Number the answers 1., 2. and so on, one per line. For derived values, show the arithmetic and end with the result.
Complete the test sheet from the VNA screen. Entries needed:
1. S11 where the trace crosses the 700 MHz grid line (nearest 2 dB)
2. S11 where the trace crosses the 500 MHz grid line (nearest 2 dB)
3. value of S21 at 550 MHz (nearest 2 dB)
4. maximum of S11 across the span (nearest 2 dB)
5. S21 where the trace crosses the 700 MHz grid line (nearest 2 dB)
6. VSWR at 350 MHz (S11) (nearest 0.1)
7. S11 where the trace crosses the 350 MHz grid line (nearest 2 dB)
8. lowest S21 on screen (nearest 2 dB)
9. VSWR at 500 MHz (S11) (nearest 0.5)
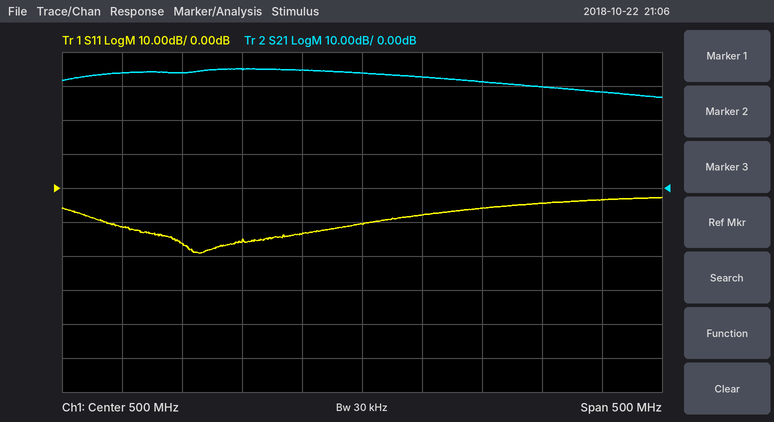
1. -4 dB
2. -10 dB
3. 32 dB
4. -2 dB
5. 28 dB
6. |Γ| = 10^(-16/20) = 0.1585; VSWR = (1 + 0.1585)/(1 − 0.1585) ≈ 1.4
7. -16 dB
8. 26 dB
9. |Γ| = 10^(-10/20) = 0.3162; VSWR = (1 + 0.3162)/(1 − 0.3162) ≈ 1.92, so 2.0 to the nearest 0.5
